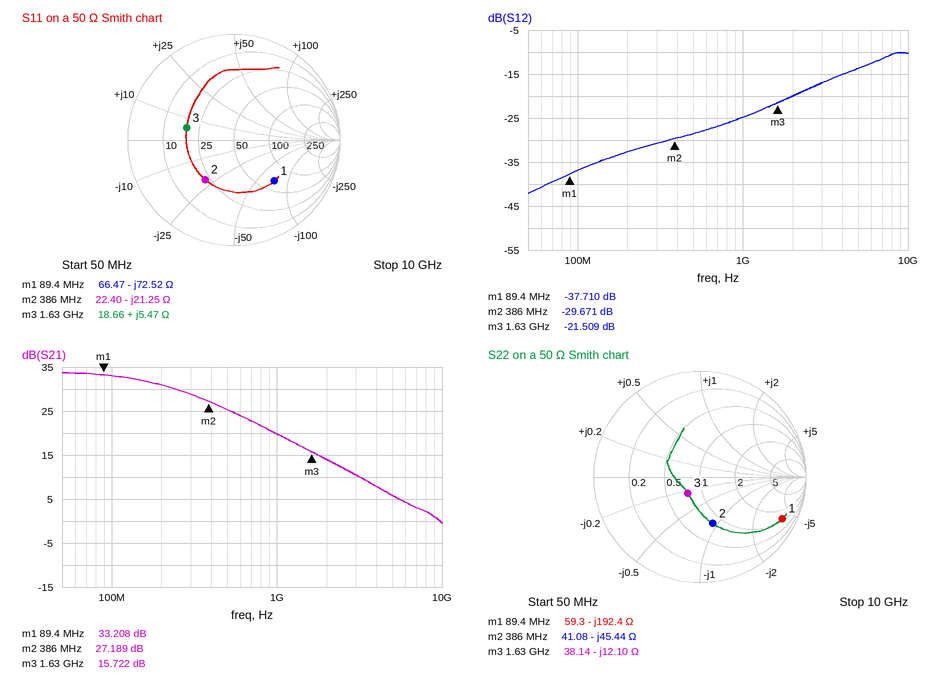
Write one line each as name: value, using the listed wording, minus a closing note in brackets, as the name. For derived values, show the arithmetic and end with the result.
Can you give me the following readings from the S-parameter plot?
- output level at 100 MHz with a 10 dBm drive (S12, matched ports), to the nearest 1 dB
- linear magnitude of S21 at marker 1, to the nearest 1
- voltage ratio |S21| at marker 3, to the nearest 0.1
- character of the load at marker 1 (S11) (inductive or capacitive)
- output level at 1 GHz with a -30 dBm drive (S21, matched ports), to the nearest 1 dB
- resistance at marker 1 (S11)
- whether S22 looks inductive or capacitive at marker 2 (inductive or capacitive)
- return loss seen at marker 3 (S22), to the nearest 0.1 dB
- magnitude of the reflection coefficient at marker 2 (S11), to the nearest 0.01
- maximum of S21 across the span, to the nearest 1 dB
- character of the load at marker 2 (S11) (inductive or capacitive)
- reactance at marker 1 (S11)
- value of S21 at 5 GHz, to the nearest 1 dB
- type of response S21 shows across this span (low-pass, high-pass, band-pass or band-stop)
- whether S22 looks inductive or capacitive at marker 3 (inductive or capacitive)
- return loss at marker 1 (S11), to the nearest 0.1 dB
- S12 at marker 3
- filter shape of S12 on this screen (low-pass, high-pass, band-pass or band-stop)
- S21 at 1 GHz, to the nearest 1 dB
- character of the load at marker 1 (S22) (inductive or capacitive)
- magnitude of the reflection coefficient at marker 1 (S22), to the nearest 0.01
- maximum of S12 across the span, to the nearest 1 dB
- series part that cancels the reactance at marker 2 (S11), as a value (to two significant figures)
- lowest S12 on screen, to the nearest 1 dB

output level at 100 MHz with a 10 dBm drive (S12, matched ports), to the nearest 1 dB: 10 dBm + (-37 dB) = -27 dBm
linear magnitude of S21 at marker 1, to the nearest 1: 10^(33.208/20) ≈ 46
voltage ratio |S21| at marker 3, to the nearest 0.1: 10^(15.722/20) ≈ 6.1
character of the load at marker 1 (S11): capacitive
output level at 1 GHz with a -30 dBm drive (S21, matched ports), to the nearest 1 dB: -30 dBm + (20 dB) = -10 dBm
resistance at marker 1: 66.47 Ω
whether S22 looks inductive or capacitive at marker 2: capacitive
return loss seen at marker 3 (S22), to the nearest 0.1 dB: 14.4 dB
magnitude of the reflection coefficient at marker 2 (S11), to the nearest 0.01: 0.46
maximum of S21 across the span, to the nearest 1 dB: 34 dB
character of the load at marker 2 (S11): capacitive
reactance at marker 1: -72.52 Ω
value of S21 at 5 GHz, to the nearest 1 dB: 6 dB
type of response S21 shows across this span: low-pass
whether S22 looks inductive or capacitive at marker 3: capacitive
return loss at marker 1 (S11), to the nearest 0.1 dB: 5.3 dB
S12 at marker 3: -21.509 dB
filter shape of S12 on this screen: high-pass
S21 at 1 GHz, to the nearest 1 dB: 20 dB
character of the load at marker 1 (S22): capacitive
magnitude of the reflection coefficient at marker 1 (S22), to the nearest 0.01: 0.87
maximum of S12 across the span, to the nearest 1 dB: -10 dB
series part that cancels the reactance at marker 2 (S11), as a value: L = 21.25 Ω/(2π × 386 MHz) ≈ 8.8 nH
lowest S12 on screen, to the nearest 1 dB: -42 dB
